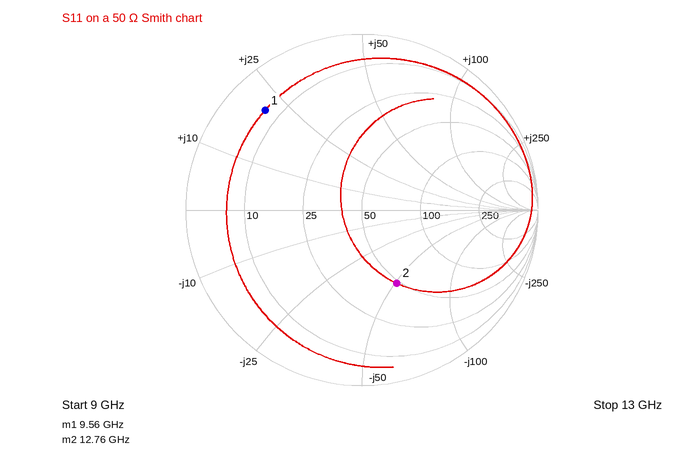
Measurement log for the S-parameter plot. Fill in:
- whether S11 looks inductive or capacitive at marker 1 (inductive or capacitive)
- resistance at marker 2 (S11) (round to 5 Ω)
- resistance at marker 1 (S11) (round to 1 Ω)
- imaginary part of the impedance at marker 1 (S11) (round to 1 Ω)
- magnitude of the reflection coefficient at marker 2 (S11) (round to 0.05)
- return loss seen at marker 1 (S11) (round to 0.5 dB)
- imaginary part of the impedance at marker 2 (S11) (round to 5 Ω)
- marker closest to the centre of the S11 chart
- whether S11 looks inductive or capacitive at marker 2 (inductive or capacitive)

inductive
50 Ω
7 Ω
+21 Ω
0.45
2.0 dB
-50 Ω
marker 2
capacitive
